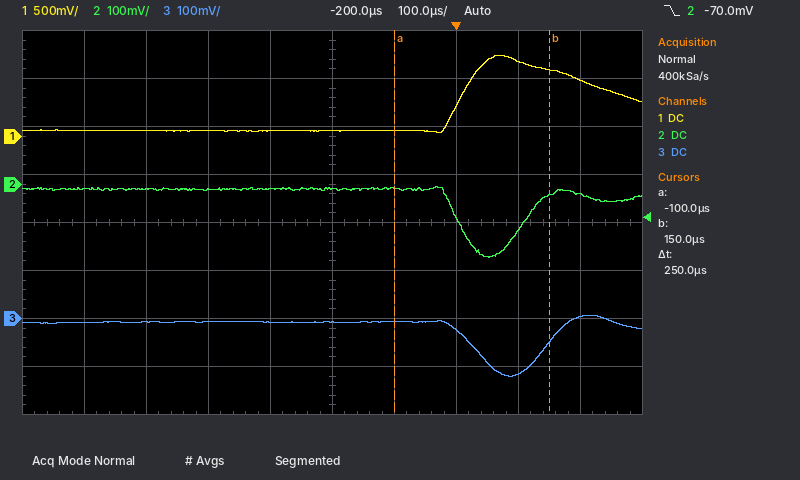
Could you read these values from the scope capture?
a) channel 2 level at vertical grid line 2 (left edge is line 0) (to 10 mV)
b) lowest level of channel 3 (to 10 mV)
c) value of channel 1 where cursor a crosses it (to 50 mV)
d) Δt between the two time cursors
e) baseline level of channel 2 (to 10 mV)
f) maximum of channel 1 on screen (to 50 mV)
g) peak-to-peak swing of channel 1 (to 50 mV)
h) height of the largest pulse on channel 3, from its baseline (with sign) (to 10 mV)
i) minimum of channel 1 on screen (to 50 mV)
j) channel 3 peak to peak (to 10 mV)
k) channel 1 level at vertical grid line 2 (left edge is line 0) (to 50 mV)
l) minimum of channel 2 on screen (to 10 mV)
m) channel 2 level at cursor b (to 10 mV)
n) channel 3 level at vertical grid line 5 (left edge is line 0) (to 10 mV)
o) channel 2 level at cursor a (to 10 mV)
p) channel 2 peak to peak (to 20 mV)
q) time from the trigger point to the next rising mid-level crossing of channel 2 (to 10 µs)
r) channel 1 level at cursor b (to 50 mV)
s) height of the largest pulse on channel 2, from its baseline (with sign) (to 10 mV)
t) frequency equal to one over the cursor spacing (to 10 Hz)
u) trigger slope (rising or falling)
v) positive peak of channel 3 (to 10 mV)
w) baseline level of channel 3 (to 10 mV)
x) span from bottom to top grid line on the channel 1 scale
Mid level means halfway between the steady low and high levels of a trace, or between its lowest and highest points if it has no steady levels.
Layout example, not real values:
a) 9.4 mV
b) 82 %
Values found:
a) -10 mV
b) -120 mV
c) 50 mV
d) 250 µs
e) -10 mV
f) 850 mV
g) 800 mV
h) -110 mV
i) 50 mV
j) 130 mV
k) 50 mV
l) -150 mV
m) -20 mV
n) -10 mV
o) -10 mV
p) 140 mV
q) 110 µs
r) 700 mV
s) -140 mV
t) 4.00 kHz
u) falling
v) 10 mV
w) -10 mV
x) 4 V
